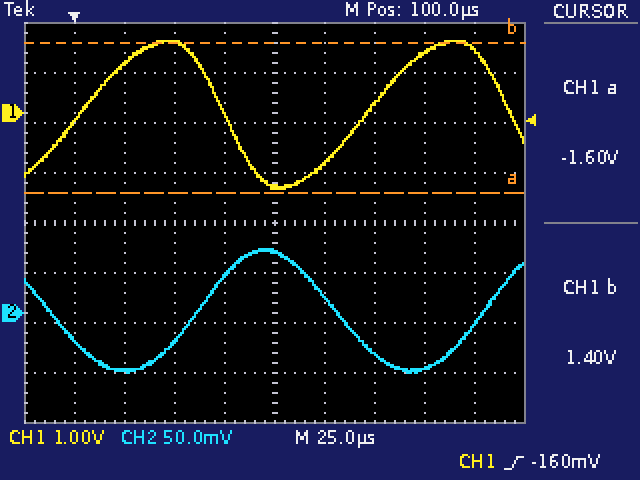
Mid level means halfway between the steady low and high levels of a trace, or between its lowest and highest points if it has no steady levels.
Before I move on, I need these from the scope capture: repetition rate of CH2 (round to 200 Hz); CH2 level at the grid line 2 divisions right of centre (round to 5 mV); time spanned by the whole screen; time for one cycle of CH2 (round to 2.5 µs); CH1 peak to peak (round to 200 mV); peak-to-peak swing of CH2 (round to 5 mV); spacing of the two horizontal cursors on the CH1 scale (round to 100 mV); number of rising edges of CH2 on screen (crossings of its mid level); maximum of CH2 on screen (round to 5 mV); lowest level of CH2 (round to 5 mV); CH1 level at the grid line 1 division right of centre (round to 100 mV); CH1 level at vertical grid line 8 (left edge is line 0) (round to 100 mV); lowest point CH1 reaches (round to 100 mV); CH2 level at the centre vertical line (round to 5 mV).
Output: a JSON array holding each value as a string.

["7.0 kHz", "-40 mV", "250 µs", "142.5 µs", "3.0 V", "125 mV", "3.0 V", "2", "65 mV", "-60 mV", "-1.0 V", "1.2 V", "-1.5 V", "60 mV"]
